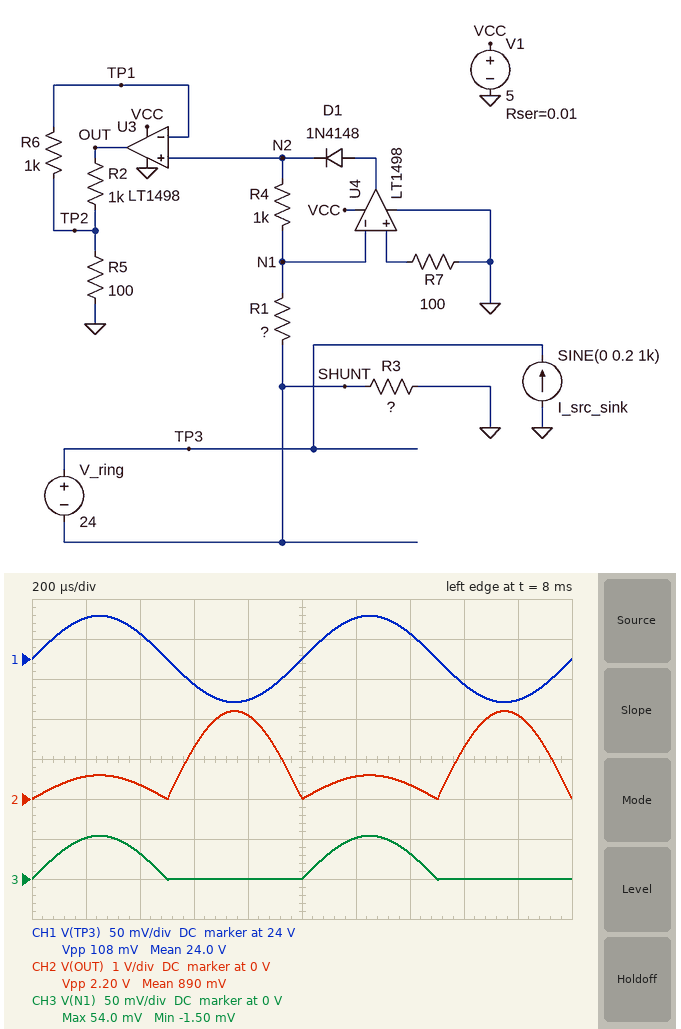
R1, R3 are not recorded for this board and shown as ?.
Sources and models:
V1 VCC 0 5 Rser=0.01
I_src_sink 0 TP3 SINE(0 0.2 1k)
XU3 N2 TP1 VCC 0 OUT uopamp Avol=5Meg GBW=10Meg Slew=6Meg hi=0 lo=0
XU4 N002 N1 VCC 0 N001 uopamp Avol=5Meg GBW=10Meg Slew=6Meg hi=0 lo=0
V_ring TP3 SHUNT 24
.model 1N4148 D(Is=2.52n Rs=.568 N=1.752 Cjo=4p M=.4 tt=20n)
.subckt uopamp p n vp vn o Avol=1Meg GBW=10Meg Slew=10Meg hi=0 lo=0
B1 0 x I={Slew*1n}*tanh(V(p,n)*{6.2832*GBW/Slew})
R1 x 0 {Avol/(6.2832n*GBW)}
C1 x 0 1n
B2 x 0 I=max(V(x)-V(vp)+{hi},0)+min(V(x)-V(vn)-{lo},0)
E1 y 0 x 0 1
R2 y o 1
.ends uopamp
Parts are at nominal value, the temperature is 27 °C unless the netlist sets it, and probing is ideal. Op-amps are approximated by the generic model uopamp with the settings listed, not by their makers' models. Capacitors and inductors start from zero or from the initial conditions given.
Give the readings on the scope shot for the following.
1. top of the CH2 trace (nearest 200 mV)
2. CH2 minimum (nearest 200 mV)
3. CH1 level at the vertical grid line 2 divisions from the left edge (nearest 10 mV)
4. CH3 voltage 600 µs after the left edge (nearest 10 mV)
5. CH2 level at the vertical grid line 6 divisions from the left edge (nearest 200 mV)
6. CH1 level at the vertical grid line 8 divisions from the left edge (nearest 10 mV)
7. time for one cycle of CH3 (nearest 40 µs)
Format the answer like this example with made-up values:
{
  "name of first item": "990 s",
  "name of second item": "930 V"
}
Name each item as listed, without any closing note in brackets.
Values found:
{
  "top of the CH2 trace": "2.2 V",
  "CH2 minimum": "0 V",
  "CH1 level at the vertical grid line 2 divisions from the left edge": "24.03 V",
  "CH3 voltage 600 µs after the left edge": "0 V",
  "CH2 level at the vertical grid line 6 divisions from the left edge": "600 mV",
  "CH1 level at the vertical grid line 8 divisions from the left edge": "23.97 V",
  "time for one cycle of CH3": "1.00 ms"
}
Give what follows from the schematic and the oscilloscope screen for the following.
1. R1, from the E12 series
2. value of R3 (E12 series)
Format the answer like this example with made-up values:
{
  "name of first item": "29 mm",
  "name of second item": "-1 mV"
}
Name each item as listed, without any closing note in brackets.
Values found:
{
  "R1, from the E12 series": "270 Ω",
  "value of R3": "0.27 Ω"
}
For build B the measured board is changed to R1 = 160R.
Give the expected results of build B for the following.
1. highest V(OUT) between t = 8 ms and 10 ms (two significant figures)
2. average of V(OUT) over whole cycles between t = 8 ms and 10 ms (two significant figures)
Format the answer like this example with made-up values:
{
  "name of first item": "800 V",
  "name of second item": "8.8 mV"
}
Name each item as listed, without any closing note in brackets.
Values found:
{
  "highest V(OUT) between t = 8 ms and 10 ms": "3.7 V",
  "average of V(OUT) over whole cycles between t = 8 ms and 10 ms": "1.4 V"
}
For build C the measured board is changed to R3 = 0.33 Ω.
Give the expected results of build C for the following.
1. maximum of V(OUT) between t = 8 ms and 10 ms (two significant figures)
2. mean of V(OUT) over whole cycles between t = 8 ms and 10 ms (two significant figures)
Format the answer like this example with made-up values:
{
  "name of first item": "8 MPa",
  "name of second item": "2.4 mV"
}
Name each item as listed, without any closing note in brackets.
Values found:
{
  "maximum of V(OUT) between t = 8 ms and 10 ms": "2.7 V",
  "mean of V(OUT) over whole cycles between t = 8 ms and 10 ms": "1.1 V"
}
